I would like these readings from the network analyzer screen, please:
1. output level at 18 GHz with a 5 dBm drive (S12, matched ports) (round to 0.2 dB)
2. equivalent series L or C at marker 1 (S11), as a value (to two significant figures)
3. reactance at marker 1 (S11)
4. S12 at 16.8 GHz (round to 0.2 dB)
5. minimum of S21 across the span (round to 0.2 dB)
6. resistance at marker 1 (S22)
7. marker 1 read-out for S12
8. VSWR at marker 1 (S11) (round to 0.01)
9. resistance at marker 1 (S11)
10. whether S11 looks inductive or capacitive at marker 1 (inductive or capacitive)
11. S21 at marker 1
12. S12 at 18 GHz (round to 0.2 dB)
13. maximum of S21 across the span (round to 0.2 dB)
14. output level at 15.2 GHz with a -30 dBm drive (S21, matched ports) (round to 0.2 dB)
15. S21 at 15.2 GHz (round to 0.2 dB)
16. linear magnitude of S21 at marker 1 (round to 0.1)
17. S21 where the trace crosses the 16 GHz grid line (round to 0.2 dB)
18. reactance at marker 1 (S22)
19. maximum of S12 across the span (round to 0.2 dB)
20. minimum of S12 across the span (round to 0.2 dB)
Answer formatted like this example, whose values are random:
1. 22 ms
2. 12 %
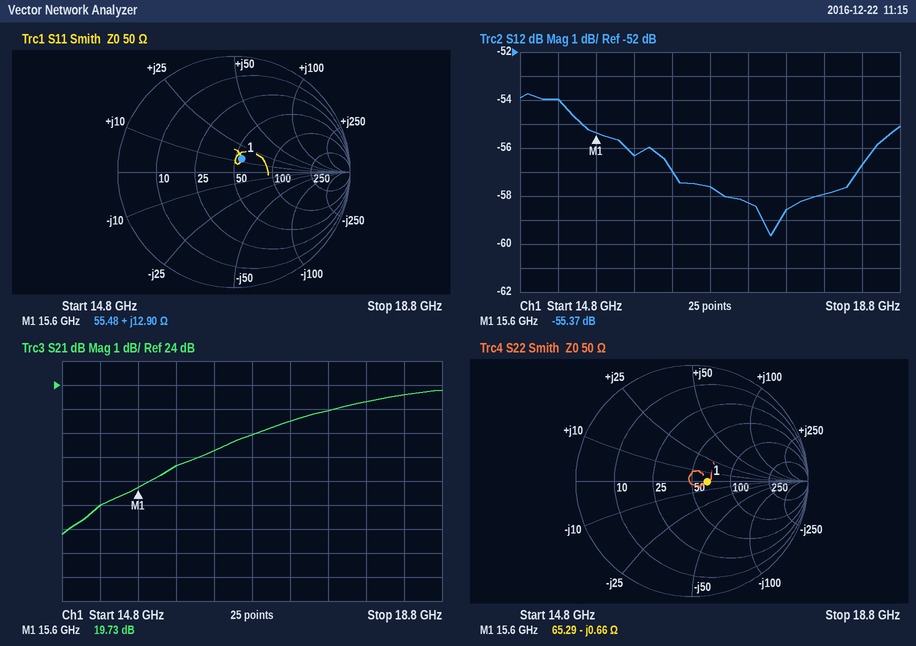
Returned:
1. -53.0 dBm
2. 130 pH
3. +12.90 Ω
4. -57.6 dB
5. 17.8 dB
6. 65.29 Ω
7. -55.37 dB
8. 1.30
9. 55.48 Ω
10. inductive
11. 19.73 dB
12. -58.0 dB
13. 23.8 dB
14. -11.0 dBm
15. 19.0 dB
16. 9.7
17. 20.6 dB
18. -0.66 Ω
19. -53.8 dB
20. -59.6 dB
